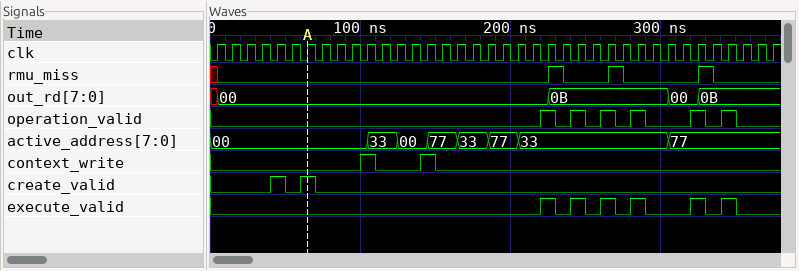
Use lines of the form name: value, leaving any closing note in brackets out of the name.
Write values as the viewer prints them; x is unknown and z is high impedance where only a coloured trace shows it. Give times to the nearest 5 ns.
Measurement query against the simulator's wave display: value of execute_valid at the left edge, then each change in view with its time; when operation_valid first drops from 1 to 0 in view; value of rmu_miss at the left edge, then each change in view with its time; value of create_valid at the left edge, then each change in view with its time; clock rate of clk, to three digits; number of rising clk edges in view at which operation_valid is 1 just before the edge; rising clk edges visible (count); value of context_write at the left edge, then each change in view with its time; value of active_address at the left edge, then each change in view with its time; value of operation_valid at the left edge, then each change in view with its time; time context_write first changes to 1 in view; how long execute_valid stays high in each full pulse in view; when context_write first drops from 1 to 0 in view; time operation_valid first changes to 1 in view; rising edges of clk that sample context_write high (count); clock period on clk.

value of execute_valid at the left edge, then each change in view with its time: 0, 1 at 220 ns, 0 at 230 ns, 1 at 240 ns, 0 at 250 ns, 1 at 260 ns, 0 at 270 ns, 1 at 280 ns, 0 at 290 ns, 1 at 320 ns, 0 at 330 ns, 1 at 340 ns, 0 at 350 ns
when operation_valid first drops from 1 to 0 in view: 230 ns
value of rmu_miss at the left edge, then each change in view with its time: x, 0 at 5 ns, 1 at 225 ns, 0 at 235 ns, 1 at 265 ns, 0 at 275 ns, 1 at 325 ns, 0 at 335 ns
value of create_valid at the left edge, then each change in view with its time: 0, 1 at 40 ns, 0 at 50 ns, 1 at 60 ns, 0 at 70 ns
clock rate of clk, to three digits: 100 MHz
number of rising clk edges in view at which operation_valid is 1 just before the edge: 6
rising clk edges visible: 38
value of context_write at the left edge, then each change in view with its time: 0, 1 at 100 ns, 0 at 110 ns, 1 at 140 ns, 0 at 150 ns
value of active_address at the left edge, then each change in view with its time: 00, 33 at 105 ns, 00 at 125 ns, 77 at 145 ns, 33 at 165 ns, 77 at 185 ns, 33 at 205 ns, 77 at 305 ns
value of operation_valid at the left edge, then each change in view with its time: 0, 1 at 220 ns, 0 at 230 ns, 1 at 240 ns, 0 at 250 ns, 1 at 260 ns, 0 at 270 ns, 1 at 280 ns, 0 at 290 ns, 1 at 320 ns, 0 at 330 ns, 1 at 340 ns, 0 at 350 ns
time context_write first changes to 1 in view: 100 ns
how long execute_valid stays high in each full pulse in view: 10 ns, 10 ns, 10 ns, 10 ns, 10 ns, 10 ns
when context_write first drops from 1 to 0 in view: 110 ns
time operation_valid first changes to 1 in view: 220 ns
rising edges of clk that sample context_write high: 2
clock period on clk: 10 ns
